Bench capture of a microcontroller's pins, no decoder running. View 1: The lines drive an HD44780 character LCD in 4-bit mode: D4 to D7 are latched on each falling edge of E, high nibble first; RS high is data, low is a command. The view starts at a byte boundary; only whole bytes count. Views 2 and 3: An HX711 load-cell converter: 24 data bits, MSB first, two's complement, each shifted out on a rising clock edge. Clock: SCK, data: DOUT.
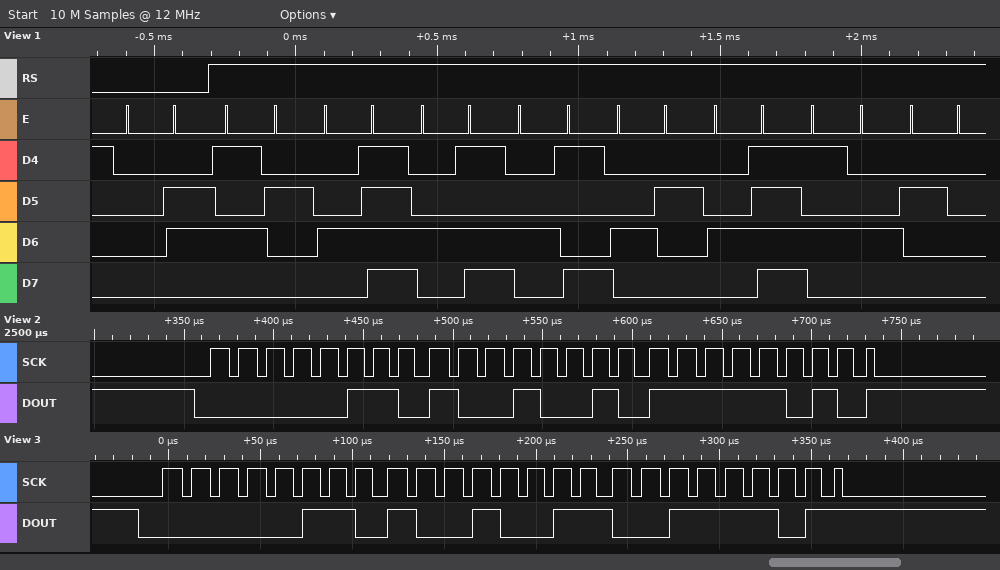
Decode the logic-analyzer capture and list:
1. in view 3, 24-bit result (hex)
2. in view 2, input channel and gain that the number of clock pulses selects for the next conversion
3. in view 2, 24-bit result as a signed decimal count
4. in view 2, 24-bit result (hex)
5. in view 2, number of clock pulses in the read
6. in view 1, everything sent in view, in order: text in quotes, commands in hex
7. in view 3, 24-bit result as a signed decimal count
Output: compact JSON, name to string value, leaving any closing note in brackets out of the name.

{"in view 3, 24-bit result": "0x06933D", "in view 2, input channel and gain that the number of clock pulses selects for the next conversion": "channel A, gain 128", "in view 2, 24-bit result as a signed decimal count": "430842", "in view 2, 24-bit result": "0x0692FA", "in view 2, number of clock pulses in the read": "25", "in view 1, everything sent in view, in order: text in quotes, commands in hex": "0x06 \"ROMIBOT \"", "in view 3, 24-bit result as a signed decimal count": "430909"}
